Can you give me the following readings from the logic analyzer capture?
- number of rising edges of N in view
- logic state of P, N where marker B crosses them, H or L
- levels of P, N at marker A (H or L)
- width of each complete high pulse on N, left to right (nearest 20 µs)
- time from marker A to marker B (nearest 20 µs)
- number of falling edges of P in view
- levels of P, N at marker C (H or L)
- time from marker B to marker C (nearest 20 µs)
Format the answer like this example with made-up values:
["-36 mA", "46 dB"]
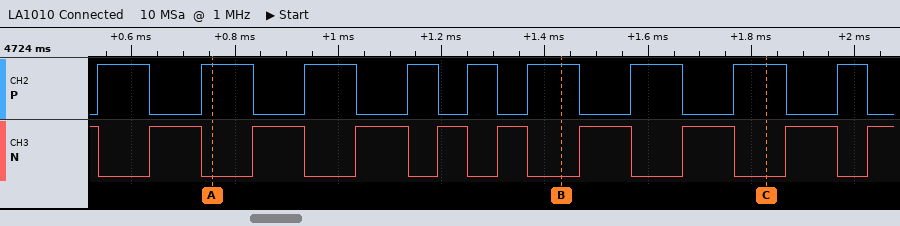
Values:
["9", "P=H, N=L", "P=H, N=L", "100 µs, 100 µs, 100 µs, 60 µs, 60 µs, 100 µs, 100 µs, 100 µs", "680 µs", "9", "P=H, N=L", "400 µs"]
